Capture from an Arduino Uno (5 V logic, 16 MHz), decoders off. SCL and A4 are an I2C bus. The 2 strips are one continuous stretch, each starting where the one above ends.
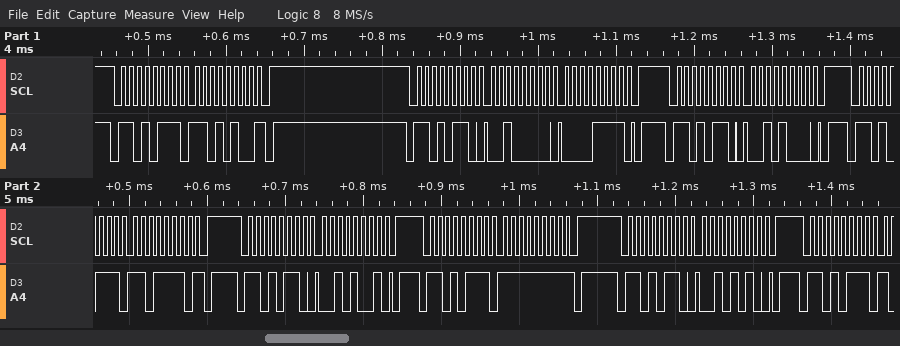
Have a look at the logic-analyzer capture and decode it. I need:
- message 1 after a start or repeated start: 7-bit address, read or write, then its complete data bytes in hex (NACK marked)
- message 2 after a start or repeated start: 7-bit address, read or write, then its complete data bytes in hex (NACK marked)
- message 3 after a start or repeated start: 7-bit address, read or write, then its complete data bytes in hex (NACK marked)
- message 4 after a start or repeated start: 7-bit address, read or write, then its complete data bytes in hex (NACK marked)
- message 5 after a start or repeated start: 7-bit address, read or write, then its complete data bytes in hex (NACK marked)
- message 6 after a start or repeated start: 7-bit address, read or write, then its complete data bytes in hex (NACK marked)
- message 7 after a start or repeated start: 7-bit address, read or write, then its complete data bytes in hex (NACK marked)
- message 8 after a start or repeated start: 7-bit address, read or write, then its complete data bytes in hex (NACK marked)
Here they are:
0x6B read: D4 NACK
0x6B write: 20 0F
0x6B write: 28
0x6B read: DE NACK
0x6B write: 29
0x6B read: FF NACK
0x6B write: 2A
0x6B read
